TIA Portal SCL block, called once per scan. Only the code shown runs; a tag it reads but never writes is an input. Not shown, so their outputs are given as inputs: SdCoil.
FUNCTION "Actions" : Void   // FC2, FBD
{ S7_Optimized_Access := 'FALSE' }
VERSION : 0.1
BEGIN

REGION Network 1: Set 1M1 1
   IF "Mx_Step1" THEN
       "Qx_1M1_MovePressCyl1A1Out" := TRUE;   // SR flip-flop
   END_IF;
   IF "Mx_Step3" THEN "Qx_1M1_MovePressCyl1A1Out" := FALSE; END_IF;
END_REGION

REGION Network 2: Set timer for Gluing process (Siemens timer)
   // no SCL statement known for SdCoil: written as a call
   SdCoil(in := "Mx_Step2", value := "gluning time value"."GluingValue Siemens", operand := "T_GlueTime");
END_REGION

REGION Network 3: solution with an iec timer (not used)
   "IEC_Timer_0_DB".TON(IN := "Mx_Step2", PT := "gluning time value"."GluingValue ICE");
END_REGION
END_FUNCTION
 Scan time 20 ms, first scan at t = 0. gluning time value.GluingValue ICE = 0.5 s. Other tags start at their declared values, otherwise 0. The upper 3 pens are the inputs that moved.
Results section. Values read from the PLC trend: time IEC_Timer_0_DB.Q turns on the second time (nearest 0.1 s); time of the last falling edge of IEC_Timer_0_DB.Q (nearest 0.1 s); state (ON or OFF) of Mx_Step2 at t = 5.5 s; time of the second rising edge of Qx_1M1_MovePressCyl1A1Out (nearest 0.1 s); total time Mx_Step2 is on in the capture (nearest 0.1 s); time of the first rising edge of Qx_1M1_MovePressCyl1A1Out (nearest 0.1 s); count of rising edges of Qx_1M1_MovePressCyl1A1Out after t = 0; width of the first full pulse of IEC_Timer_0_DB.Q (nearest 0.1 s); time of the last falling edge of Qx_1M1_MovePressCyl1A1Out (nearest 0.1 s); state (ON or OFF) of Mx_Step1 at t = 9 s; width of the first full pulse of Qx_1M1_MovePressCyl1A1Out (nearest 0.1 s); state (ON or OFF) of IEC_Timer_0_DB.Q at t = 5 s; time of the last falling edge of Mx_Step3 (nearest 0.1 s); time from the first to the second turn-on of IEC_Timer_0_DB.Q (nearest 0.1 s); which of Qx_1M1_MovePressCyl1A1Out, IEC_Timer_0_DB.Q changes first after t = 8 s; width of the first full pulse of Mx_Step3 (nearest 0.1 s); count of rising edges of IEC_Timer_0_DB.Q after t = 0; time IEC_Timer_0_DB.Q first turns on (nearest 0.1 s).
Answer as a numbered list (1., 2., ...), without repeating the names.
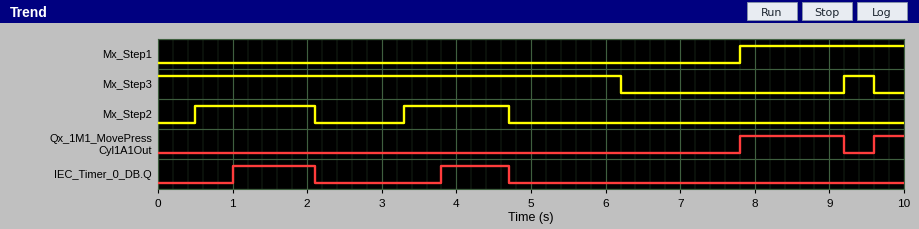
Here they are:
1. 3.8 s
2. 4.7 s
3. OFF
4. 9.6 s
5. 3.0 s
6. 7.8 s
7. 2
8. 1.1 s
9. 9.2 s
10. ON
11. 1.4 s
12. OFF
13. 9.6 s
14. 2.8 s
15. Qx_1M1_MovePressCyl1A1Out
16. 0.4 s
17. 2
18. 1.0 s
